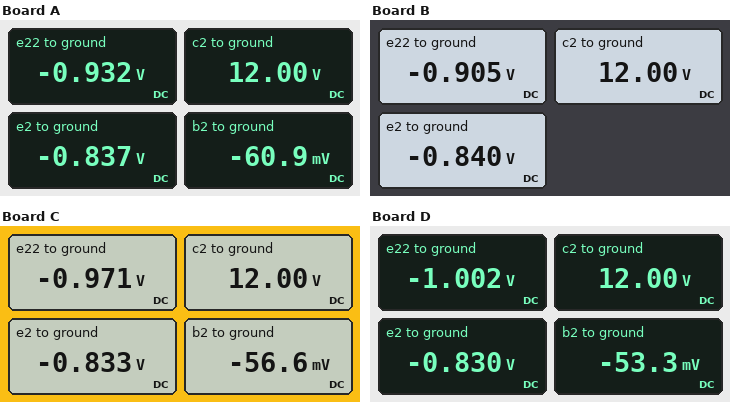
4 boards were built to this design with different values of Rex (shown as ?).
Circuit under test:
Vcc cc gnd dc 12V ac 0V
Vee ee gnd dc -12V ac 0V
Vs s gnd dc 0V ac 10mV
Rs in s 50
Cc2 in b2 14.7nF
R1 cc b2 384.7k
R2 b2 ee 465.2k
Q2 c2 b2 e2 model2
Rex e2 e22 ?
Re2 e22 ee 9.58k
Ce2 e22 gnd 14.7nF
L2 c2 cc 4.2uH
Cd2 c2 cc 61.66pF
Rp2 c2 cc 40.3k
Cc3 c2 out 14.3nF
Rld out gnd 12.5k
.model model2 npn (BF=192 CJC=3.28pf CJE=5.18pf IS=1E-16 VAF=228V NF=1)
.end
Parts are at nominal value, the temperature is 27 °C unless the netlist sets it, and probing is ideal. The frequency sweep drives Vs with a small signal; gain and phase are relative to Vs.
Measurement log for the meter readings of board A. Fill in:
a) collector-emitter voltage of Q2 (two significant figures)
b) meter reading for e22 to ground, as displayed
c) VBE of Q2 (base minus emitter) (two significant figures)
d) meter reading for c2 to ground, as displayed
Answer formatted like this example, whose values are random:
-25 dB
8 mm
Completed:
13 V
-0.932 V
780 mV
12.00 V
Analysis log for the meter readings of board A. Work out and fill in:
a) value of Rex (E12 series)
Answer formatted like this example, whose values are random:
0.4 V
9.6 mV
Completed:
82 Ω
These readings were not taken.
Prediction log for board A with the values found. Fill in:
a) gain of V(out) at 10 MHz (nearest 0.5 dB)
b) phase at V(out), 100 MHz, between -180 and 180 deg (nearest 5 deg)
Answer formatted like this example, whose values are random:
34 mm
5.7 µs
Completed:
32.5 dB
75 deg
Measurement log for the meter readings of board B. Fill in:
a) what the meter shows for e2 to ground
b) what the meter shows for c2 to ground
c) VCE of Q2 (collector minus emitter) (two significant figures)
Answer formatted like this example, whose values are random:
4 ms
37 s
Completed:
-0.840 V
12.00 V
13 V
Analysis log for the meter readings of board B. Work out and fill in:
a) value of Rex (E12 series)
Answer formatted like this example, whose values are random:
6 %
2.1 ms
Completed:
56 Ω
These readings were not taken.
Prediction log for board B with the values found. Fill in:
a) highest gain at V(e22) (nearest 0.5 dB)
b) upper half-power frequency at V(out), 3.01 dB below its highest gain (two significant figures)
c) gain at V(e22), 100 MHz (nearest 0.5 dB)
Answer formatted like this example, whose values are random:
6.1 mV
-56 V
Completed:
0 dB
9.9 MHz
-57.5 dB
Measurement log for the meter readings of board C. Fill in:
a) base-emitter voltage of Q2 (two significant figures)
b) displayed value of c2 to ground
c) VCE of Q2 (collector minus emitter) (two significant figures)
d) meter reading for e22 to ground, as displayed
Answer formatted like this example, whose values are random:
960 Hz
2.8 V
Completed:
780 mV
12.00 V
13 V
-0.971 V
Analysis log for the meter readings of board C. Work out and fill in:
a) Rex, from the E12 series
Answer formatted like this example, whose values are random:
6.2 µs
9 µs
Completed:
120 Ω
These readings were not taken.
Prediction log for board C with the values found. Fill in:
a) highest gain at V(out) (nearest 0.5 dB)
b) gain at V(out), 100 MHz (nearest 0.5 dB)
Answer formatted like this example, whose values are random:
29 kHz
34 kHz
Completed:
36.5 dB
-15.0 dB
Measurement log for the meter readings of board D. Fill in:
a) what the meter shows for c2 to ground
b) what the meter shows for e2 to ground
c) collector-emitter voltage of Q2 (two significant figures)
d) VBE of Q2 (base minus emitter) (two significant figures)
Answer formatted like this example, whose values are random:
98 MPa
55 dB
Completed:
12.00 V
-0.830 V
13 V
780 mV
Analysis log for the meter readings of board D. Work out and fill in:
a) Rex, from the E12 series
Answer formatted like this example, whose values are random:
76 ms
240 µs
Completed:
150 Ω
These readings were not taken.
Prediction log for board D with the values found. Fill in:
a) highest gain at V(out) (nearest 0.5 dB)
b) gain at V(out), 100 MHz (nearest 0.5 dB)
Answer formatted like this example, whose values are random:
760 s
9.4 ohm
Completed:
34.5 dB
-16.5 dB
